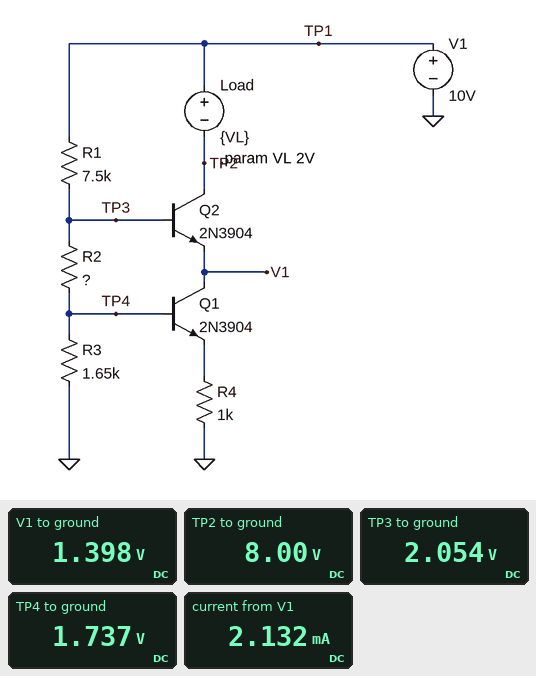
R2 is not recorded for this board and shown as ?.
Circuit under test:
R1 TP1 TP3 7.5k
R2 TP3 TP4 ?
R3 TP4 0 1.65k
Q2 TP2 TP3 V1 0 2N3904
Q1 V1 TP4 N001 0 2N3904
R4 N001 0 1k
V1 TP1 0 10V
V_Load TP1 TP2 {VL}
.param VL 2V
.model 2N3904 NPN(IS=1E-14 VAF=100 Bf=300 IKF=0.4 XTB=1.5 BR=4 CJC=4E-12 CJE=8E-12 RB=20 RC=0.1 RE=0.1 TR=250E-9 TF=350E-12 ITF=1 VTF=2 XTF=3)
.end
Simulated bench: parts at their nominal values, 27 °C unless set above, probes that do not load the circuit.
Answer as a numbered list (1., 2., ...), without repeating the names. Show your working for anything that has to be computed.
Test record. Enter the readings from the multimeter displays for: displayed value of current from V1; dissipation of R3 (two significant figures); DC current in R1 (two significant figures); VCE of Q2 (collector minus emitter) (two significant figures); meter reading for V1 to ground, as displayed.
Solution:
1. 2.132 mA
2. (1.737 V)^2 / 1.65 kΩ = 1.8 mW
3. (10 V - 2.054 V) / 7.5 kΩ = 1.1 mA
4. 8 V - 1.398 V = 6.6 V
5. 1.398 V
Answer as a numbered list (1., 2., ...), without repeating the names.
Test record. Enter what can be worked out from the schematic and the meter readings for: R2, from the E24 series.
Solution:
1. 300 Ω
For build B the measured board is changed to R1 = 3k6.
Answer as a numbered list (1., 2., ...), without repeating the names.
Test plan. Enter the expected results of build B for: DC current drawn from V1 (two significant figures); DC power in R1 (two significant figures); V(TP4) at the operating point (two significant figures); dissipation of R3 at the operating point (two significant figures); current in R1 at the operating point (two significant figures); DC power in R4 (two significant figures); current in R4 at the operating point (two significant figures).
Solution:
1. 4.1 mA
2. 12 mW
3. 3.0 V
4. 5.3 mW
5. 1.8 mA
6. 5.2 mW
7. 2.3 mA
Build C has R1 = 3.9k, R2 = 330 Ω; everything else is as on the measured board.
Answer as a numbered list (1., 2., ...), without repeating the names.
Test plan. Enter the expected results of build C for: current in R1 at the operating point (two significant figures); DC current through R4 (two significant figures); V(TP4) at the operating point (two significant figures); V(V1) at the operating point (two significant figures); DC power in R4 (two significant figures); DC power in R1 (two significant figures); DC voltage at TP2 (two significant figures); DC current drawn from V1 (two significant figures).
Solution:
1. 1.7 mA
2. 2.1 mA
3. 2.8 V
4. 2.7 V
5. 4.5 mW
6. 11 mW
7. 8.0 V
8. 3.8 mA
